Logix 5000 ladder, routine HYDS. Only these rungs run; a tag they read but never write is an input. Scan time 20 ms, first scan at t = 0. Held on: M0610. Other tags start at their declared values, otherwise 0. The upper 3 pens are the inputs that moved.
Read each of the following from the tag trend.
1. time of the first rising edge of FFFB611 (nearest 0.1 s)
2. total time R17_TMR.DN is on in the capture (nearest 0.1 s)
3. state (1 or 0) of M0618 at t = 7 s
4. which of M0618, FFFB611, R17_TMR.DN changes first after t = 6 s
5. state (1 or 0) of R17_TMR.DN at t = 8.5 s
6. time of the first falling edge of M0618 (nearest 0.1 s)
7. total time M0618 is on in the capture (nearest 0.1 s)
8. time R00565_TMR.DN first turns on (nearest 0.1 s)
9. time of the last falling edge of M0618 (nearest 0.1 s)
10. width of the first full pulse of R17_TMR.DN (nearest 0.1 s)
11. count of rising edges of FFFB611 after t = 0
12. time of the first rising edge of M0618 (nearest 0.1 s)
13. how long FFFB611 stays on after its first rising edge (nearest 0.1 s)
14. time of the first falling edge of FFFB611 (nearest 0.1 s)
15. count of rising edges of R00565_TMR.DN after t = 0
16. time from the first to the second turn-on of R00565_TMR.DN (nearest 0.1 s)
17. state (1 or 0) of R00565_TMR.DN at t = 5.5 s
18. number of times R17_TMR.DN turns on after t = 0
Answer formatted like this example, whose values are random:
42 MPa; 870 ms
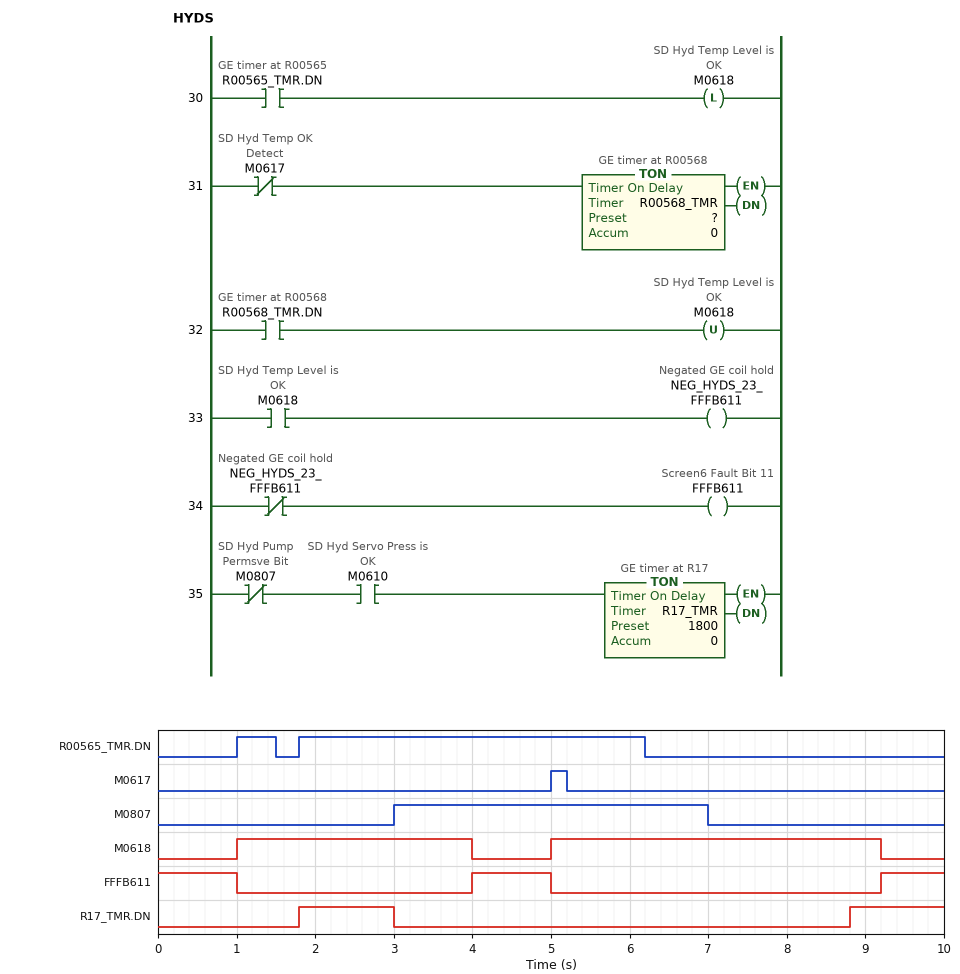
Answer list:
4.0 s; 2.4 s; 1; R17_TMR.DN; 0; 4.0 s; 7.2 s; 1.0 s; 9.2 s; 1.2 s; 2; 1.0 s; 1.0 s; 1.0 s; 2; 0.8 s; 1; 2
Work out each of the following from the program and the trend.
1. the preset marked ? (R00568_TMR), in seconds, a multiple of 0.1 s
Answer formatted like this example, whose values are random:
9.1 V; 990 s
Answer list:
4.0 s
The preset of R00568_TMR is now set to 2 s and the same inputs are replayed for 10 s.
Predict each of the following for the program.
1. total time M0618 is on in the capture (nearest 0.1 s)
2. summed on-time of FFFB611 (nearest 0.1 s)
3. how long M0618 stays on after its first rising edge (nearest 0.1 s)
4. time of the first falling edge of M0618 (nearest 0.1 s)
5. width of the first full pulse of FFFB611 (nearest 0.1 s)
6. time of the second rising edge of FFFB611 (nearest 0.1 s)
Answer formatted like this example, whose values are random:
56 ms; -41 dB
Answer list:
3.2 s; 6.8 s; 1.0 s; 2.0 s; 3.0 s; 7.2 s
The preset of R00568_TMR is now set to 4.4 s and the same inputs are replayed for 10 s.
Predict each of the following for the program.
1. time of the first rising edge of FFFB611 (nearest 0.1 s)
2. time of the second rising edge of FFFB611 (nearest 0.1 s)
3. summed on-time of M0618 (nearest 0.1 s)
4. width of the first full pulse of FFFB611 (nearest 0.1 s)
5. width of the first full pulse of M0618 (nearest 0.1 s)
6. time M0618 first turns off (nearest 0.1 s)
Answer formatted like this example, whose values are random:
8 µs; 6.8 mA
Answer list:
4.4 s; 9.6 s; 8.0 s; 0.6 s; 3.4 s; 4.4 s
